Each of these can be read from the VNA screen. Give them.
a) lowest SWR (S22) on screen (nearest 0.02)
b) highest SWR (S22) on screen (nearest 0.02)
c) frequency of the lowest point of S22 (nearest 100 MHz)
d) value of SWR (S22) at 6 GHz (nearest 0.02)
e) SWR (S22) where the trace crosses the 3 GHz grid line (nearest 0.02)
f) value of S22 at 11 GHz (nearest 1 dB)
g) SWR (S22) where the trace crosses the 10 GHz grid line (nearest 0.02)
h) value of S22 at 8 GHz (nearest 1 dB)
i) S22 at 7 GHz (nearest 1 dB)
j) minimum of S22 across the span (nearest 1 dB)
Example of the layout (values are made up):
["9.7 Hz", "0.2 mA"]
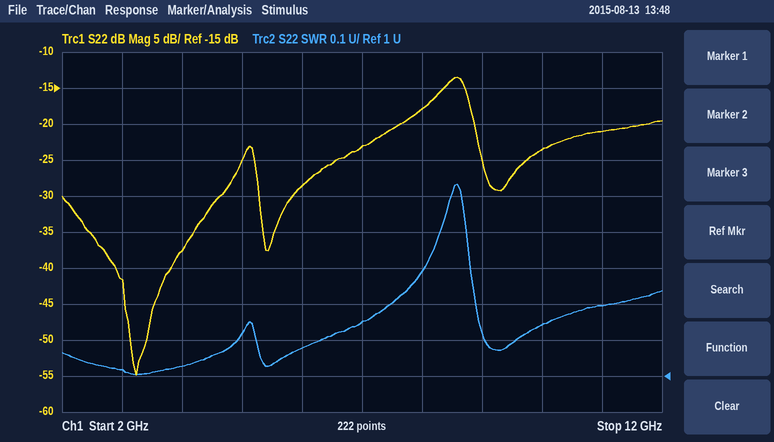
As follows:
["1.00", "1.54", "3.2 GHz", "1.08", "1.02", "-21 dB", "1.14", "-18 dB", "-23 dB", "-55 dB"]
